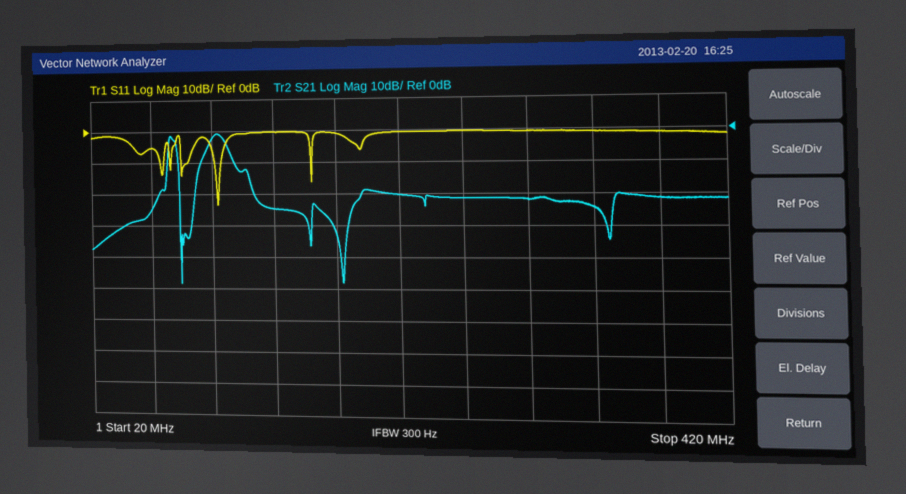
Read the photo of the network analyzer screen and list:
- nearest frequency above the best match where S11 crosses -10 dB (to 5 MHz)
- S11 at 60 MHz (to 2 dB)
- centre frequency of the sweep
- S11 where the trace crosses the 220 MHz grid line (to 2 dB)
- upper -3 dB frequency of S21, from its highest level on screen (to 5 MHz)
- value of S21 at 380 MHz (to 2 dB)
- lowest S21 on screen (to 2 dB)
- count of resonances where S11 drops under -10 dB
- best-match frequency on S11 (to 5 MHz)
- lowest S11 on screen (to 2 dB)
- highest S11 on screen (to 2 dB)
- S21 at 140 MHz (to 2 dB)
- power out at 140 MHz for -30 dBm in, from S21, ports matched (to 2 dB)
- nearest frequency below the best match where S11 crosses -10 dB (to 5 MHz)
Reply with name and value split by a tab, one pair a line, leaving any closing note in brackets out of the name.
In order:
nearest frequency above the best match where S11 crosses -10 dB	105 MHz
S11 at 60 MHz	-6 dB
centre frequency of the sweep	220 MHz
S11 where the trace crosses the 220 MHz grid line	0 dB
upper -3 dB frequency of S21, from its highest level on screen	110 MHz
value of S21 at 380 MHz	-22 dB
lowest S21 on screen	-48 dB
count of resonances where S11 drops under -10 dB	5
best-match frequency on S11	105 MHz
lowest S11 on screen	-24 dB
highest S11 on screen	0 dB
S21 at 140 MHz	-24 dB
power out at 140 MHz for -30 dBm in, from S21, ports matched	-54 dBm
nearest frequency below the best match where S11 crosses -10 dB	100 MHz
